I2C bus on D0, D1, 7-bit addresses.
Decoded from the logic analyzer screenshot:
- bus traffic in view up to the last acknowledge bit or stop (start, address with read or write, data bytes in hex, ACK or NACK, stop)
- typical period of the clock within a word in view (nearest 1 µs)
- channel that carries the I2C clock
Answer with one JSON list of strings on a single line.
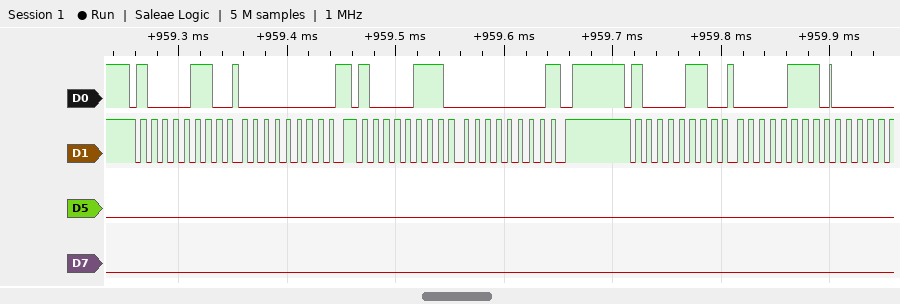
["start, address 43 write ACK, 00 ACK, repeated start, address 43 read ACK, 00 NACK, stop, start, address 43 write ACK, 07 ACK", "10 µs", "D1"]
